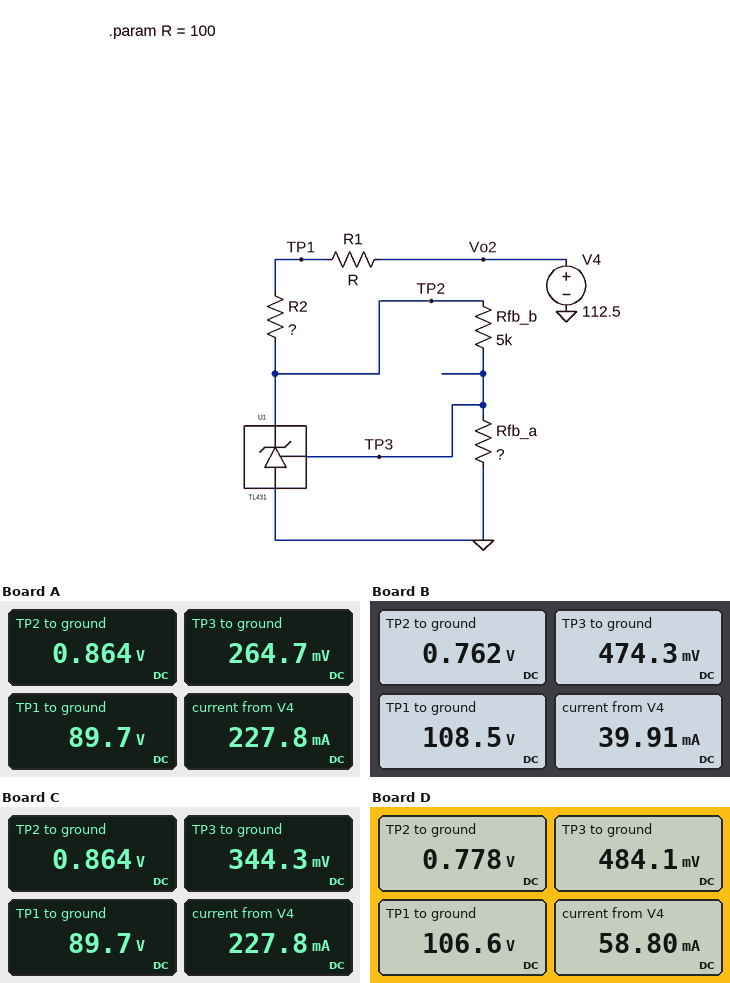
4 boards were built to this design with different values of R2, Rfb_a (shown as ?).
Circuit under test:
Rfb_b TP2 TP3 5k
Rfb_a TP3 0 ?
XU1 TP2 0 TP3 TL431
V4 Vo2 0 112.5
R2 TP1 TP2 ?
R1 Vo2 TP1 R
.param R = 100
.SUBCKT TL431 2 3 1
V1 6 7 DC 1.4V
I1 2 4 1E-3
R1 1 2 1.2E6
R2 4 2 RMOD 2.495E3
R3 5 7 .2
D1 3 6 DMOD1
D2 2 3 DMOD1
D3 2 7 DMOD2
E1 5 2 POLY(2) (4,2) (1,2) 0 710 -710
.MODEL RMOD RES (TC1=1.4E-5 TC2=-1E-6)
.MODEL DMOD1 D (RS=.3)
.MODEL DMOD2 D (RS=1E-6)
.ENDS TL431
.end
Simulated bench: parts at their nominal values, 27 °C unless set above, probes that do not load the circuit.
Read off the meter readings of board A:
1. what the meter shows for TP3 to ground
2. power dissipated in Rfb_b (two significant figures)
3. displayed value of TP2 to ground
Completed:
264.7 mV
72 µW
0.864 V
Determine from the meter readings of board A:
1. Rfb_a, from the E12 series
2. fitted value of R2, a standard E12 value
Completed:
2.2 kΩ
390 Ω
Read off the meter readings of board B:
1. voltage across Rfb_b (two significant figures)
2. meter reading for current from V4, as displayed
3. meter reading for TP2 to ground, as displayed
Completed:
290 mV
39.91 mA
0.762 V
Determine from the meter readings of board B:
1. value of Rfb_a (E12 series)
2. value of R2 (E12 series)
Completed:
8.2 kΩ
2.7 kΩ
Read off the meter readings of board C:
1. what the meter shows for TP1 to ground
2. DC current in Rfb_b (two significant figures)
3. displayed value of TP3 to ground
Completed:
89.7 V
100 µA
344.3 mV
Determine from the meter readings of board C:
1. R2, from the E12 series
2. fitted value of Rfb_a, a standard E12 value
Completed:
390 Ω
3.3 kΩ
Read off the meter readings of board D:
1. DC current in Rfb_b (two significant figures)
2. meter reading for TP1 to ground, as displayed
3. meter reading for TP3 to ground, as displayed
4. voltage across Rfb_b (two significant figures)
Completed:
59 µA
106.6 V
484.1 mV
290 mV
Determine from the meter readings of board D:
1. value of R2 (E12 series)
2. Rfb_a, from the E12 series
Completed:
1.8 kΩ
8.2 kΩ
